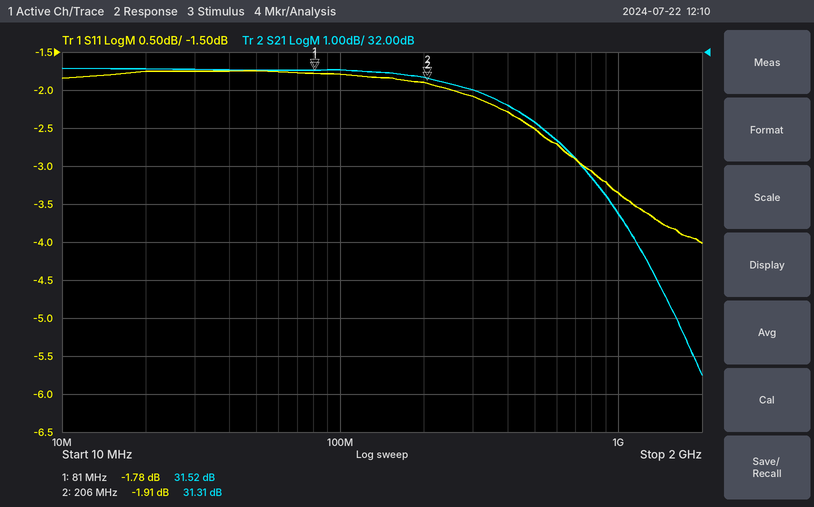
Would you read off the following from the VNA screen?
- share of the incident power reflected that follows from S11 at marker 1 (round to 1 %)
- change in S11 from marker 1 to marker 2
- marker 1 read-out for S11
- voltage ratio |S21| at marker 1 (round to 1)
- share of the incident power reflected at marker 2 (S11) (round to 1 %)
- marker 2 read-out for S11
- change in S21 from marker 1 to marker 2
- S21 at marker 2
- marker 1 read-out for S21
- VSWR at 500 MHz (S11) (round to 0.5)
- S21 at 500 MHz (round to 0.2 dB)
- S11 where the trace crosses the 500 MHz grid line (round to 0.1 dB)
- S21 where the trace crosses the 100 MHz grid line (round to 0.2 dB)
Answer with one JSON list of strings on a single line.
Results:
["66 %", "-0.13 dB", "-1.78 dB", "38", "64 %", "-1.91 dB", "-0.21 dB", "31.31 dB", "31.52 dB", "7.0", "30.2 dB", "-2.5 dB", "31.6 dB"]
